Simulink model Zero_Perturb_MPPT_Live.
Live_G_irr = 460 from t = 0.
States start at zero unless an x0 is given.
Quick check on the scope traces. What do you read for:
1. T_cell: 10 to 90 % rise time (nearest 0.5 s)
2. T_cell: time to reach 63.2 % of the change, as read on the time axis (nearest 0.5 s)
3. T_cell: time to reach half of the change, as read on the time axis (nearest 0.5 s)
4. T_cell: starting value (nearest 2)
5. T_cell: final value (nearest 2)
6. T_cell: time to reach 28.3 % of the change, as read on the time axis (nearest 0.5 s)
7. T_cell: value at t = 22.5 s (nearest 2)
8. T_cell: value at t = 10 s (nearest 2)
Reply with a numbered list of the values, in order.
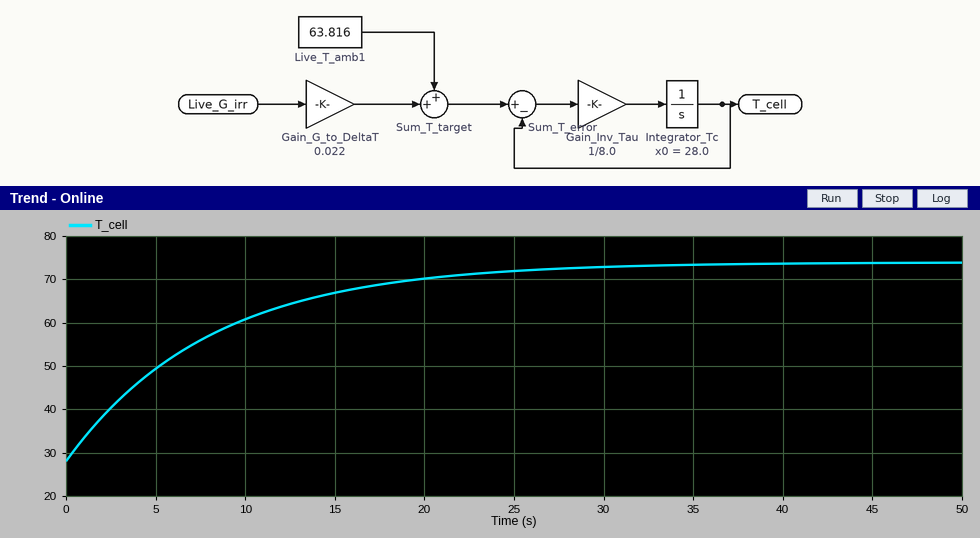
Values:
1. 17.5 s
2. 8.0 s
3. 5.5 s
4. 28
5. 74
6. 2.5 s
7. 72
8. 60
